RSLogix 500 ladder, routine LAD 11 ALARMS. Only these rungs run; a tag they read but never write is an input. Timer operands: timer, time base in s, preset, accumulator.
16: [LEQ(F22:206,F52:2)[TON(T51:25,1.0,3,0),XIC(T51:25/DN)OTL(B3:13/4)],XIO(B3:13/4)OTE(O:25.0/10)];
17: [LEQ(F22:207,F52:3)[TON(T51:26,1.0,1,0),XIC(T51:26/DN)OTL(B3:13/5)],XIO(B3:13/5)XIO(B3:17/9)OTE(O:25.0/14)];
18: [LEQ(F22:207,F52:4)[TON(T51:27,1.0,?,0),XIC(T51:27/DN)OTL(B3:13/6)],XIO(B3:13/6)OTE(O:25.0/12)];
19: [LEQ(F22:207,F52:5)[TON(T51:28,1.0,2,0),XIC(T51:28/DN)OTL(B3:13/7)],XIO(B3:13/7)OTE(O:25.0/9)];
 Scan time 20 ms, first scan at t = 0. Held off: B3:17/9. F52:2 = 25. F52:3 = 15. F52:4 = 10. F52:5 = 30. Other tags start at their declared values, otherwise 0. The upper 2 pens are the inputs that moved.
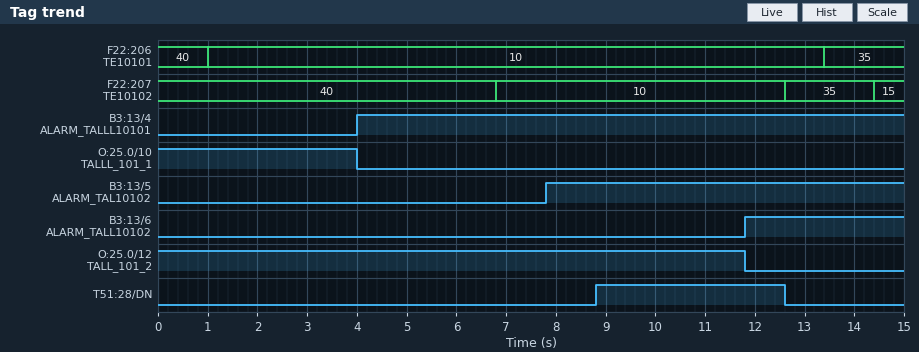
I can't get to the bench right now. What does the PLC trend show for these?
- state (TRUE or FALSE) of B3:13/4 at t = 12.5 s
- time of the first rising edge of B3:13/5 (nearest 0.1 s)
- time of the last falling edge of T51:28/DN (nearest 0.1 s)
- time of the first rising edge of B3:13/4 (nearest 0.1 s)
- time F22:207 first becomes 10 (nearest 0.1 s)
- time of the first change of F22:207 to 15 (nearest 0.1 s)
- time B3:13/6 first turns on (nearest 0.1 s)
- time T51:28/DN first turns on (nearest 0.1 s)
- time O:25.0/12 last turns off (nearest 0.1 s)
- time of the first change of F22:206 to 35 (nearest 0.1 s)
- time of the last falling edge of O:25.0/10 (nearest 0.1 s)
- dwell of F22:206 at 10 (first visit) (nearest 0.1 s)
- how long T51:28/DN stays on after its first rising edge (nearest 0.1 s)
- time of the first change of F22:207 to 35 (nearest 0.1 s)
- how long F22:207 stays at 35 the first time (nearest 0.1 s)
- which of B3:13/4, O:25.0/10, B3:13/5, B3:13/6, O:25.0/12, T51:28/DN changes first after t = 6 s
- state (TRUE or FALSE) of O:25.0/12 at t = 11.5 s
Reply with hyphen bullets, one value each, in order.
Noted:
- TRUE
- 7.8 s
- 12.6 s
- 4.0 s
- 6.8 s
- 14.4 s
- 11.8 s
- 8.8 s
- 11.8 s
- 13.4 s
- 4.0 s
- 12.4 s
- 3.8 s
- 12.6 s
- 1.8 s
- B3:13/5
- TRUE
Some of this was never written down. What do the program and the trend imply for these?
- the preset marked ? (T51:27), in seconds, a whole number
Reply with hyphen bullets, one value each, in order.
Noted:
- 5 s
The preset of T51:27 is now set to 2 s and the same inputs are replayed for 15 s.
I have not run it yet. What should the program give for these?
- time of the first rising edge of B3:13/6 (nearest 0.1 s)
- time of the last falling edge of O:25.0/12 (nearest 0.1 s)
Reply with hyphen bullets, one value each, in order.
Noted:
- 8.8 s
- 8.8 s
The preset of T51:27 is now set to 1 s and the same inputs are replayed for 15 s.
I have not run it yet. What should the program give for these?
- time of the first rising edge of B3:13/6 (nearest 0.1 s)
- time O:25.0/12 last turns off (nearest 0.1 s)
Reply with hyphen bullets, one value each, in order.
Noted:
- 7.8 s
- 7.8 s
